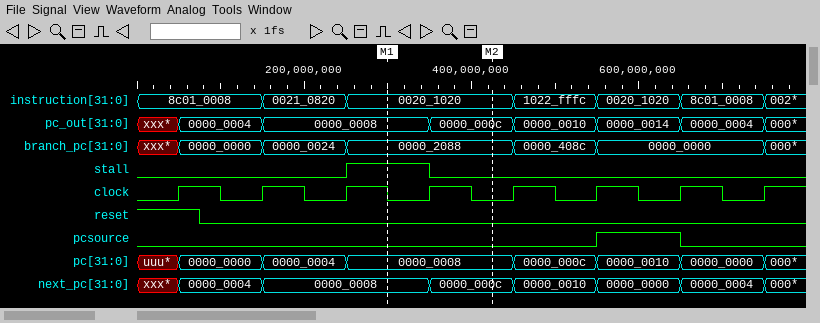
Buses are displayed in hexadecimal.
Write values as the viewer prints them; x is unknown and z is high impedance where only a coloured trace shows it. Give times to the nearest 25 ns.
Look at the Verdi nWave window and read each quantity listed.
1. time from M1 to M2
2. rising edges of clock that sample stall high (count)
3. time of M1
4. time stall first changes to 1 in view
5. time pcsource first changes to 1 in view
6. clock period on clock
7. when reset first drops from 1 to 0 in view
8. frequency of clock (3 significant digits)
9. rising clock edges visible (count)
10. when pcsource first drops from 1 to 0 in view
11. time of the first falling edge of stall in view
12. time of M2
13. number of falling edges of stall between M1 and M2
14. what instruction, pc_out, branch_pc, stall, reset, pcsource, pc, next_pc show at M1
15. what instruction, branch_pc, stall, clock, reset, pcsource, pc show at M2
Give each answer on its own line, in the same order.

125 ns
1
300 ns
250 ns
550 ns
100 ns
75 ns
10.0 MHz
8
650 ns
350 ns
425 ns
1
instruction=0020_1020, pc_out=0000_0008, branch_pc=0000_2088, stall=1, reset=0, pcsource=0, pc=0000_0008, next_pc=0000_0008
instruction=0020_1020, branch_pc=0000_2088, stall=0, clock=0, reset=0, pcsource=0, pc=0000_0008
